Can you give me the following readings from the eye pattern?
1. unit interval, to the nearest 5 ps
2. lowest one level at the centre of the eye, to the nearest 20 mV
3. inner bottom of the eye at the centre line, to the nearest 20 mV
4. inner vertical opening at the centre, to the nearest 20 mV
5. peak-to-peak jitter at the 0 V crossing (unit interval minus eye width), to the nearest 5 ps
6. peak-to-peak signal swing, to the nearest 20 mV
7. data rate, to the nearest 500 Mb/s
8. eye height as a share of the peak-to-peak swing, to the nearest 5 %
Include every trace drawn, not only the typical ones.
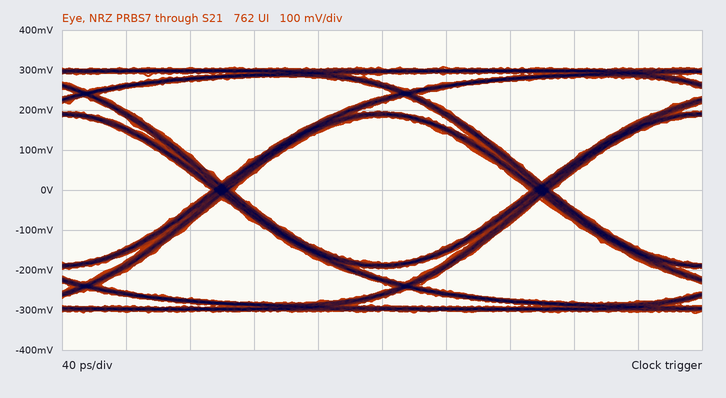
200 ps
180 mV
-180 mV
360 mV
15 ps
620 mV
5.0 Gb/s
60 %
